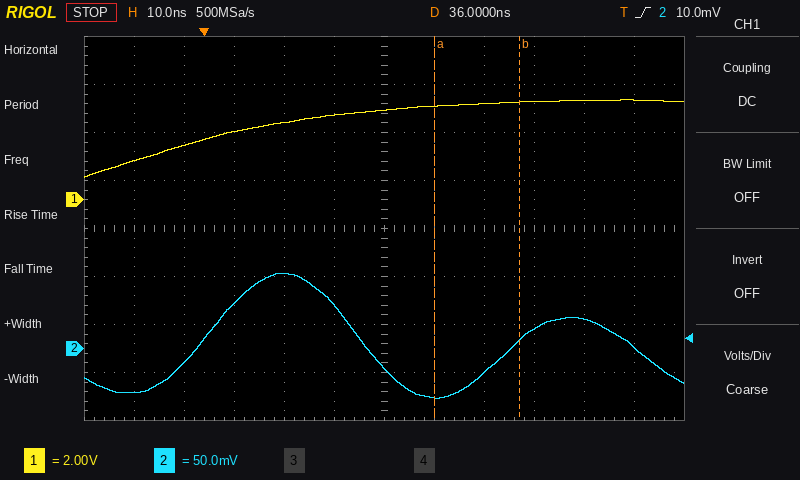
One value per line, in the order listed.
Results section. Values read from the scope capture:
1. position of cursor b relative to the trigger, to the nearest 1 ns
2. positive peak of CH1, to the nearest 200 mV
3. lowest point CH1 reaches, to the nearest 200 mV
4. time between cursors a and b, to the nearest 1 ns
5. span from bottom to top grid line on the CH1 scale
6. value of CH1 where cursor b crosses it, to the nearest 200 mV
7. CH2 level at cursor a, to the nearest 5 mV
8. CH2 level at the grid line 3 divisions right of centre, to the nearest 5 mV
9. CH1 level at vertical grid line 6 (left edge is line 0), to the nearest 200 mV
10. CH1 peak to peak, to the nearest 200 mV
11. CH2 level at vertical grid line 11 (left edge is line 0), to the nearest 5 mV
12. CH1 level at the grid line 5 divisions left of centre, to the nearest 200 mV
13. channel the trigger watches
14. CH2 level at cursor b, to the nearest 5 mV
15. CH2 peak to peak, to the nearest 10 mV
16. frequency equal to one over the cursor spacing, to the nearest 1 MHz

+63 ns
4.2 V
1.0 V
17 ns
16 V
4.0 V
-50 mV
20 mV
3.8 V
3.2 V
0 mV
1.6 V
CH2
10 mV
130 mV
59 MHz
